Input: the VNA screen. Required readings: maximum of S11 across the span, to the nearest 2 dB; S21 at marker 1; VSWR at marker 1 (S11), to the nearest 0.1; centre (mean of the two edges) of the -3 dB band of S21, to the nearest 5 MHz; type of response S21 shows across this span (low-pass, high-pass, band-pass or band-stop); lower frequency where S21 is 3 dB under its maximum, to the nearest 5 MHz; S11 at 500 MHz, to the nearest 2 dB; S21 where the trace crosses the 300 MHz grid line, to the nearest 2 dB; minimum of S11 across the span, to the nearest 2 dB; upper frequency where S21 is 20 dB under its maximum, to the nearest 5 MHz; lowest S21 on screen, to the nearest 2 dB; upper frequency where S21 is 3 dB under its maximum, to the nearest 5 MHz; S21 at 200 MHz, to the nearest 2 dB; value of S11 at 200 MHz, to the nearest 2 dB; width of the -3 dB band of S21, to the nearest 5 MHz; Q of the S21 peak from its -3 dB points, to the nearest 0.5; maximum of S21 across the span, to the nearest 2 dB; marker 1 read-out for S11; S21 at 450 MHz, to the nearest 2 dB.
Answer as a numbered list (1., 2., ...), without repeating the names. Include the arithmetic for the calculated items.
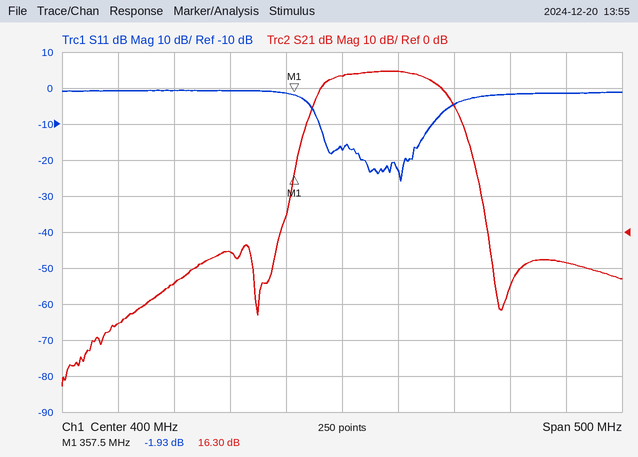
1. 0 dB
2. 16.30 dB
3. (1 + 0.8008)/(1 − 0.8008) ≈ 9.0
4. 435 MHz
5. band-pass
6. 385 MHz
7. -4 dB
8. -6 dB
9. -26 dB
10. 515 MHz
11. -42 dB
12. 480 MHz
13. -26 dB
14. 0 dB
15. 480 MHz − 385 MHz = 95 MHz
16. 432.5 MHz / 95 MHz ≈ 4.5
17. 44 dB
18. -1.93 dB
19. 44 dB
